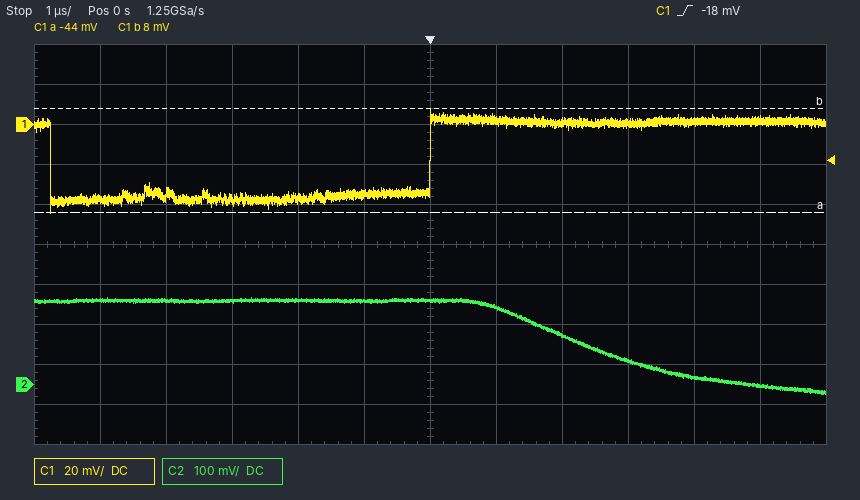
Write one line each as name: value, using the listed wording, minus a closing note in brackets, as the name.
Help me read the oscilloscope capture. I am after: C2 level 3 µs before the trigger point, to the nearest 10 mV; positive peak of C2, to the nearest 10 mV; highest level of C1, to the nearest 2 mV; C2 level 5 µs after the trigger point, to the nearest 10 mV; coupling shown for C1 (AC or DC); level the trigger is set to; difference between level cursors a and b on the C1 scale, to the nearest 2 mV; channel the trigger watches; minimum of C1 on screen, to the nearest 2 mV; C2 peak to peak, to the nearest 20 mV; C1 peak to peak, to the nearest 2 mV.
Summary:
C2 level 3 µs before the trigger point, to the nearest 10 mV: 210 mV
positive peak of C2, to the nearest 10 mV: 220 mV
highest level of C1, to the nearest 2 mV: 8 mV
C2 level 5 µs after the trigger point, to the nearest 10 mV: 0 mV
coupling shown for C1: DC
level the trigger is set to: -18 mV
difference between level cursors a and b on the C1 scale, to the nearest 2 mV: 52 mV
channel the trigger watches: C1
minimum of C1 on screen, to the nearest 2 mV: -44 mV
C2 peak to peak, to the nearest 20 mV: 240 mV
C1 peak to peak, to the nearest 2 mV: 52 mV
